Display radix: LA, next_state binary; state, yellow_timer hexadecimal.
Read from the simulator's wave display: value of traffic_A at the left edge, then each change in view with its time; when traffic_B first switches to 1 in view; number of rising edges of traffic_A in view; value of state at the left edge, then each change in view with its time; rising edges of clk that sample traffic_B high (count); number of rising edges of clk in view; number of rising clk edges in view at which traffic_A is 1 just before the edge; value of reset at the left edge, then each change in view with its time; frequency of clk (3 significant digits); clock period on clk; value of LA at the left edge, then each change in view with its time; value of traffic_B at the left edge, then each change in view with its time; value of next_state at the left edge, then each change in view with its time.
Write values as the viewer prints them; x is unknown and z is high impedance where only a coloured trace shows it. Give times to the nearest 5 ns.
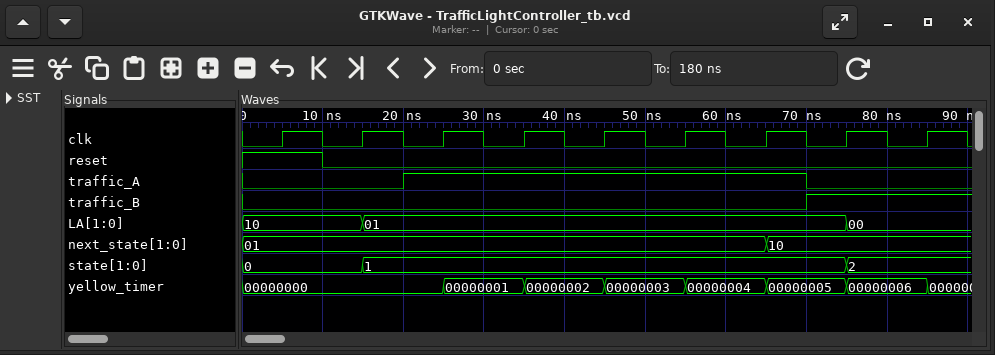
0, 1 at 20 ns, 0 at 70 ns
70 ns
1
0, 1 at 15 ns, 2 at 75 ns
2
9
5
1, 0 at 10 ns
100 MHz
10 ns
10, 01 at 15 ns, 00 at 75 ns
0, 1 at 70 ns
01, 10 at 65 ns
